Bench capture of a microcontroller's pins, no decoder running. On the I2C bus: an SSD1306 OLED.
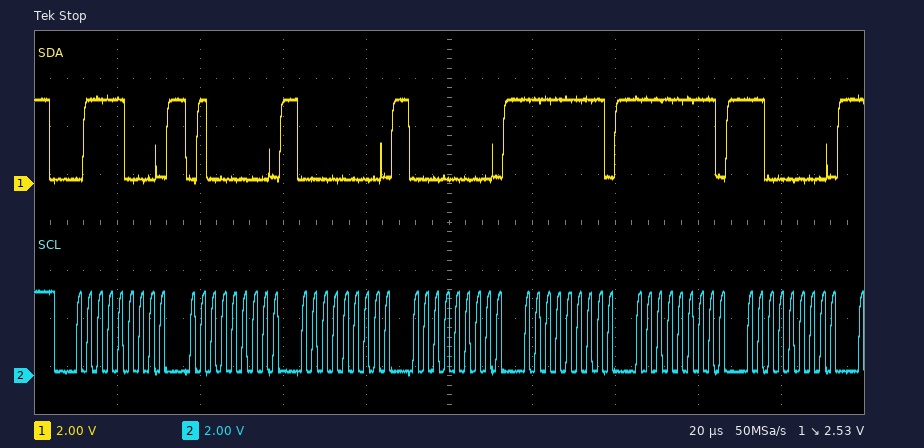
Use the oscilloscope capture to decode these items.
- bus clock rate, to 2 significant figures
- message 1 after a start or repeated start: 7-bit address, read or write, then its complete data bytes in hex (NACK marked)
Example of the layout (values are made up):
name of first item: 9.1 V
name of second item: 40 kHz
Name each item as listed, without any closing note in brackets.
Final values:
bus clock rate, to 2 significant figures: 400 kHz
message 1 after a start or repeated start: 7-bit address, read or write, then its complete data bytes in hex: 0x3C write: 40 00 00 FF FF C0
